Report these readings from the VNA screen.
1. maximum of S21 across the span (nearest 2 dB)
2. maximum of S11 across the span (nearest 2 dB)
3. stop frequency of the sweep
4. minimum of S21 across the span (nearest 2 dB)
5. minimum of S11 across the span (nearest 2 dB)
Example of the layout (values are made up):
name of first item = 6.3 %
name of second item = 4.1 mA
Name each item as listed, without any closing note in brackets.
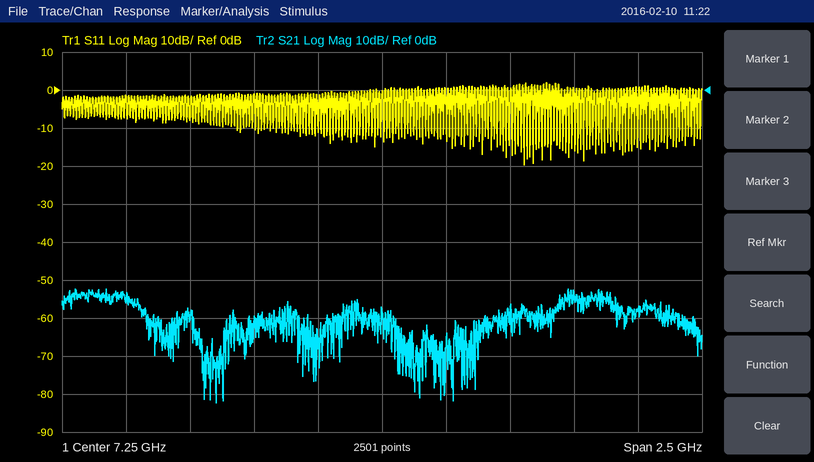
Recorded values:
maximum of S21 across the span = -52 dB
maximum of S11 across the span = 2 dB
stop frequency of the sweep = 8.5 GHz
minimum of S21 across the span = -82 dB
minimum of S11 across the span = -20 dB
